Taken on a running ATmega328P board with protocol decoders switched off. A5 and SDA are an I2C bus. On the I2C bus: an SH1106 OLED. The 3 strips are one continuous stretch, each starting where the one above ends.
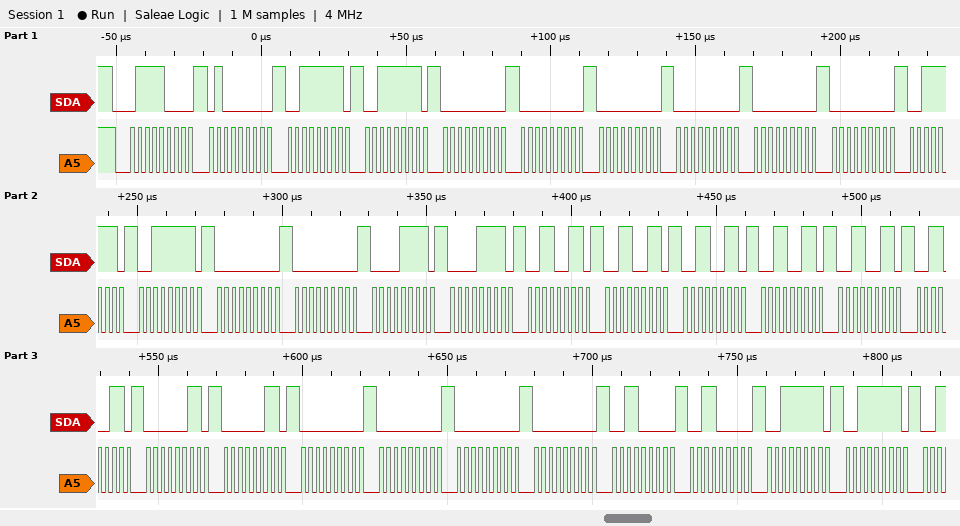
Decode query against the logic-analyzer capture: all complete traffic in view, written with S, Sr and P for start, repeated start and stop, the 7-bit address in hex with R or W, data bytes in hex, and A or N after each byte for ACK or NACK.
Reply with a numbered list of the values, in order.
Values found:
1. S 3CW A 40 A 3F A 3F A 00 A 00 A 00 A 00 A 00 A 00 A 3F A 3F A 00 A 00 A 0F A 0F A 33 A 33 A 33 A 33 A 33 A 33 A 03 A 03 A 00 A 00 A 00 A 00 A 30 A 30 A 3F A 3F A
